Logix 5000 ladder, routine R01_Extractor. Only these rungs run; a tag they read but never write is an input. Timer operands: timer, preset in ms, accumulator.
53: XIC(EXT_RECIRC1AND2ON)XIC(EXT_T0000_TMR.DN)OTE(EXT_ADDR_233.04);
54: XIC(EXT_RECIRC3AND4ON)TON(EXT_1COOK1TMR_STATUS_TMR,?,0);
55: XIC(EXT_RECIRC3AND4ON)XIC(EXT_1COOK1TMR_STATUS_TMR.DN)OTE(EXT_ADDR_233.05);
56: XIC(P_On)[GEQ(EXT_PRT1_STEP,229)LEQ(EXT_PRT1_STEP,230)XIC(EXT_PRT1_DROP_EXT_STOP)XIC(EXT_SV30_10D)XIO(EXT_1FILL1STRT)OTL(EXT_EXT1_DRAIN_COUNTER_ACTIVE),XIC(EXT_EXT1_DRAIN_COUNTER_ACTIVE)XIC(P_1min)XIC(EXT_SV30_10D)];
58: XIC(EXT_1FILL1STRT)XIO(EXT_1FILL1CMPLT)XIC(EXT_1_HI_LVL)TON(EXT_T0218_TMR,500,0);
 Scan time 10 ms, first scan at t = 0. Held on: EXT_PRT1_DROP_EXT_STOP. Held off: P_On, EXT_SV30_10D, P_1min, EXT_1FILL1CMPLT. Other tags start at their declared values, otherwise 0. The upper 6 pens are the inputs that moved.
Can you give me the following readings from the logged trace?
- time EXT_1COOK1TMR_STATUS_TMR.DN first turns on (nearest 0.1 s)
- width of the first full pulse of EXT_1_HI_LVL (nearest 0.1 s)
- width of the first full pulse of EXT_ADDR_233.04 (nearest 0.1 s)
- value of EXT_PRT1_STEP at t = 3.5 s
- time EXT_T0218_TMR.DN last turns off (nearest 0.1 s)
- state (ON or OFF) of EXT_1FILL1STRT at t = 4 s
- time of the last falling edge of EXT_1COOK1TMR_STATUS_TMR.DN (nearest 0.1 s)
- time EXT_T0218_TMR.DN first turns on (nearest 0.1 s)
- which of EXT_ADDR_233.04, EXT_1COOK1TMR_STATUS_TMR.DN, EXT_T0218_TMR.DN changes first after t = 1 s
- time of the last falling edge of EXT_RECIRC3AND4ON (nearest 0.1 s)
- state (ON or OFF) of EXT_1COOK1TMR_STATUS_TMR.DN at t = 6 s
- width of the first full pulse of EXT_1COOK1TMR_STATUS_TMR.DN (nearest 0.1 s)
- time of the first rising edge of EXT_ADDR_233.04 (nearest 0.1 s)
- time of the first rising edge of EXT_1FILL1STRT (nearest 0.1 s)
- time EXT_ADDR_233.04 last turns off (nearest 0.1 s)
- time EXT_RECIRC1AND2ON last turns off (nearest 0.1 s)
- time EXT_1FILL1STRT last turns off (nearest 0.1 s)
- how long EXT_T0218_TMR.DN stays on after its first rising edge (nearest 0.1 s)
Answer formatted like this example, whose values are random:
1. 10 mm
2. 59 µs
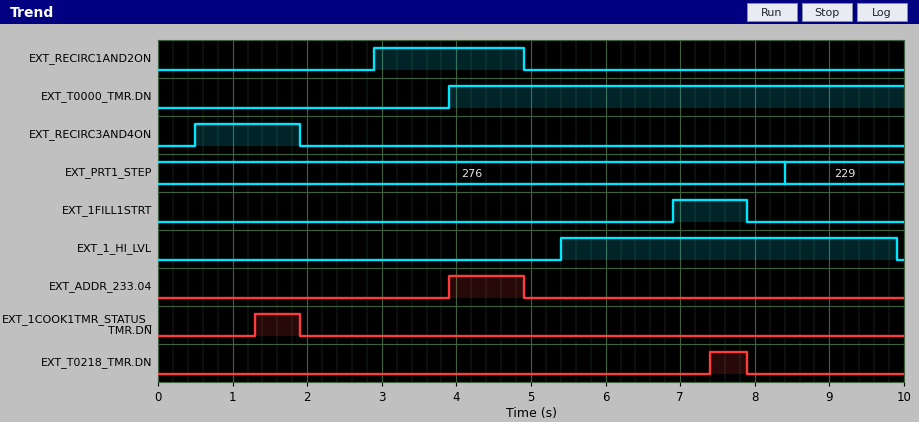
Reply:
1. 1.3 s
2. 4.5 s
3. 1.0 s
4. 276
5. 7.9 s
6. OFF
7. 1.9 s
8. 7.4 s
9. EXT_1COOK1TMR_STATUS_TMR.DN
10. 1.9 s
11. OFF
12. 0.6 s
13. 3.9 s
14. 6.9 s
15. 4.9 s
16. 4.9 s
17. 7.9 s
18. 0.5 s
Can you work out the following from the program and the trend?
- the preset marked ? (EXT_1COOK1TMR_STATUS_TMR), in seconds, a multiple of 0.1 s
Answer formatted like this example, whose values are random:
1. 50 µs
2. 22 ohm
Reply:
1. 0.8 s
